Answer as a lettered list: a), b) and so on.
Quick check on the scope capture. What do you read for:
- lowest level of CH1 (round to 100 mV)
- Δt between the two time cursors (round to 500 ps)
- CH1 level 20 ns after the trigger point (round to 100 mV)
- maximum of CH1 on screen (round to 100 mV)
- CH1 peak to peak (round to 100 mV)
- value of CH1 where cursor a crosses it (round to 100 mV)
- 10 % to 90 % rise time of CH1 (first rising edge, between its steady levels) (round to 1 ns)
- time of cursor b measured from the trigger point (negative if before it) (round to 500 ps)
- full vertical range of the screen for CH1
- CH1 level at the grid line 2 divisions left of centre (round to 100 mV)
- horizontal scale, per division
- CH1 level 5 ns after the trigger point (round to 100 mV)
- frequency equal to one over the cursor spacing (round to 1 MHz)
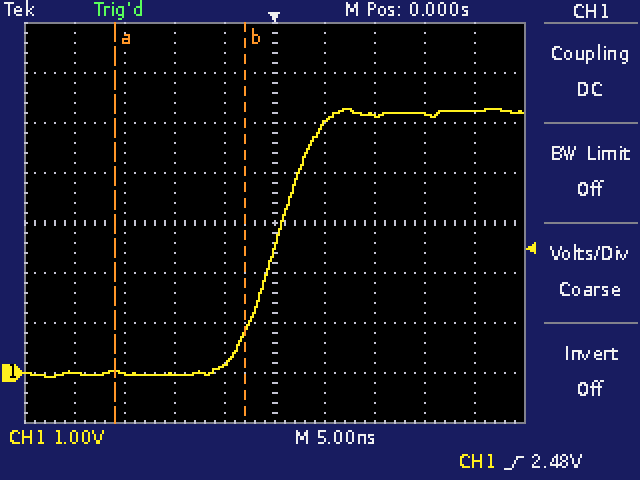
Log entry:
a) -100 mV
b) 13.0 ns
c) 5.2 V
d) 5.3 V
e) 5.4 V
f) 0.0 V
g) 8 ns
h) -3.0 ns
i) 8 V
j) 0.0 V
k) 5 ns
l) 5.0 V
m) 77 MHz
